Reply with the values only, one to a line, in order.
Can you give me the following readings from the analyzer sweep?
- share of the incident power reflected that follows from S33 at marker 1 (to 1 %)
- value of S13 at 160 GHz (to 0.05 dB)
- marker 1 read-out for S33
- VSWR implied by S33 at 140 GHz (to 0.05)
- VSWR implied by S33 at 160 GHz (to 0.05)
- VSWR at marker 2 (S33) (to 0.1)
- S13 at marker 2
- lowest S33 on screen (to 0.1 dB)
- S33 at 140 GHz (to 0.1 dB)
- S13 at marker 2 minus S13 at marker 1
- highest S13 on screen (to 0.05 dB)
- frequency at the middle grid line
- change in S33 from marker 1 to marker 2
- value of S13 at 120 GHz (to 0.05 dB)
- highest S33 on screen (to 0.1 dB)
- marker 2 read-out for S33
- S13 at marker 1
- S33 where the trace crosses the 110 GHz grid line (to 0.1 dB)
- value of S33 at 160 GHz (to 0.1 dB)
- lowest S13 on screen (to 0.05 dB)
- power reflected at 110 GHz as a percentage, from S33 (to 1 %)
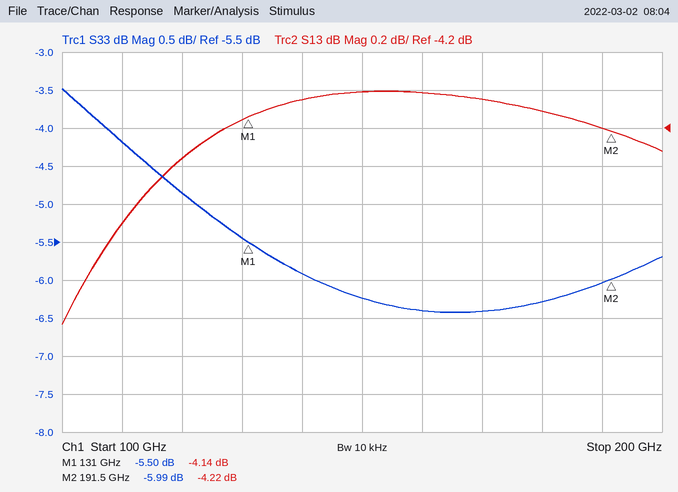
28 %
-4.00 dB
-5.50 dB
3.05
2.85
3.0
-4.22 dB
-6.4 dB
-5.9 dB
-0.08 dB
-4.00 dB
150 GHz
-0.49 dB
-4.35 dB
-3.5 dB
-5.99 dB
-4.14 dB
-4.2 dB
-6.4 dB
-5.25 dB
38 %
